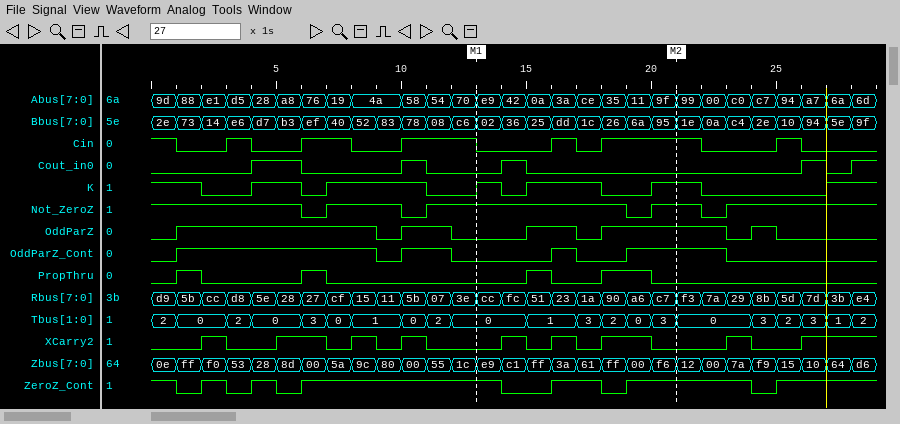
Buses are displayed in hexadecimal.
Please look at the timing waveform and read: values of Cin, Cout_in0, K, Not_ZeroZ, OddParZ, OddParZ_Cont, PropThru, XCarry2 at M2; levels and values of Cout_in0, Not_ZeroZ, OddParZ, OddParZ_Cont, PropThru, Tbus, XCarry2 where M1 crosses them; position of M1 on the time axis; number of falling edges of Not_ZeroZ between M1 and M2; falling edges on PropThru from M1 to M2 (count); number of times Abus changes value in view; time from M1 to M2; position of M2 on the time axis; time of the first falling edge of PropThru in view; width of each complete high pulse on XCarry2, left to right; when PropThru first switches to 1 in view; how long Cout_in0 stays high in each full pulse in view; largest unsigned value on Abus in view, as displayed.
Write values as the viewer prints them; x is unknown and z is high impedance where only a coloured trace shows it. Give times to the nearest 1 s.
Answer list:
Cin=1, Cout_in0=0, K=1, Not_ZeroZ=1, OddParZ=1, OddParZ_Cont=1, PropThru=0, XCarry2=0
Cout_in0=0, Not_ZeroZ=1, OddParZ=0, OddParZ_Cont=0, PropThru=0, Tbus=0, XCarry2=0
13 s
1
2
27
8 s
21 s
2 s
1 s, 2 s, 1 s, 1 s, 1 s, 1 s, 2 s, 1 s
1 s
2 s, 1 s, 1 s, 1 s
e9
